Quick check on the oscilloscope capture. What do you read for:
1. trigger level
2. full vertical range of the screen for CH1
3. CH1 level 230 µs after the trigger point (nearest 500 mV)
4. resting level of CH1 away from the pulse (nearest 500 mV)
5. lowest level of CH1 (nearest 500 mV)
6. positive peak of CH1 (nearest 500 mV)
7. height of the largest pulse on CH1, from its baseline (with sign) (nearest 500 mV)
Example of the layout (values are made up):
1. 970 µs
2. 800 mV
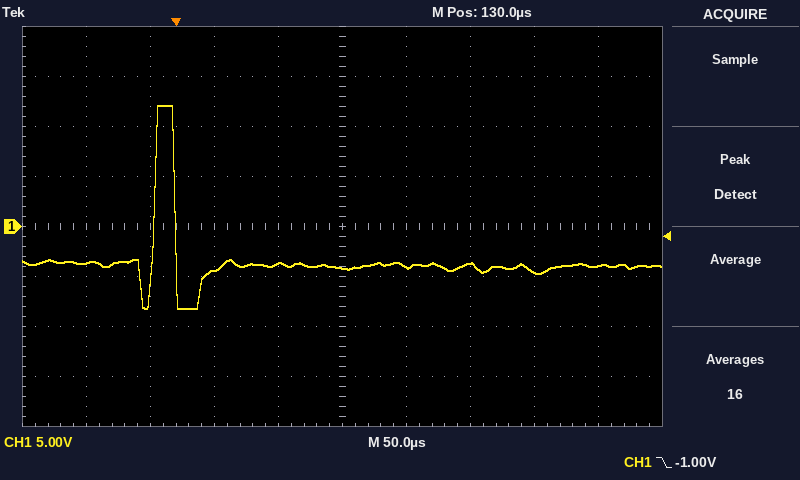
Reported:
1. -1.00 V
2. 40 V
3. -3.5 V
4. -4.0 V
5. -8.0 V
6. 12.0 V
7. +16.0 V
